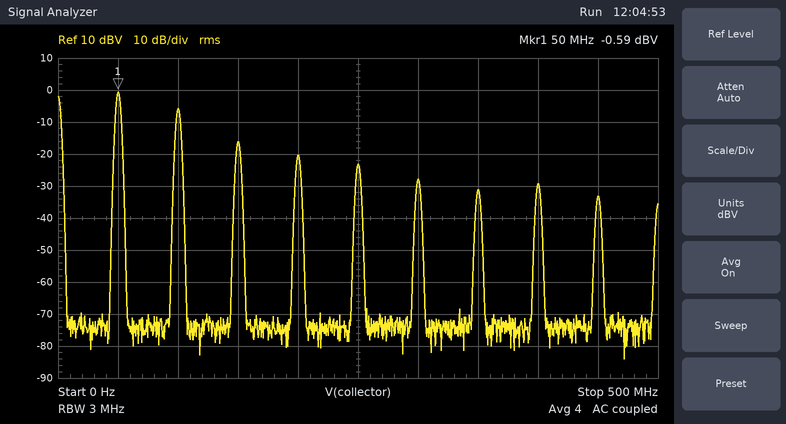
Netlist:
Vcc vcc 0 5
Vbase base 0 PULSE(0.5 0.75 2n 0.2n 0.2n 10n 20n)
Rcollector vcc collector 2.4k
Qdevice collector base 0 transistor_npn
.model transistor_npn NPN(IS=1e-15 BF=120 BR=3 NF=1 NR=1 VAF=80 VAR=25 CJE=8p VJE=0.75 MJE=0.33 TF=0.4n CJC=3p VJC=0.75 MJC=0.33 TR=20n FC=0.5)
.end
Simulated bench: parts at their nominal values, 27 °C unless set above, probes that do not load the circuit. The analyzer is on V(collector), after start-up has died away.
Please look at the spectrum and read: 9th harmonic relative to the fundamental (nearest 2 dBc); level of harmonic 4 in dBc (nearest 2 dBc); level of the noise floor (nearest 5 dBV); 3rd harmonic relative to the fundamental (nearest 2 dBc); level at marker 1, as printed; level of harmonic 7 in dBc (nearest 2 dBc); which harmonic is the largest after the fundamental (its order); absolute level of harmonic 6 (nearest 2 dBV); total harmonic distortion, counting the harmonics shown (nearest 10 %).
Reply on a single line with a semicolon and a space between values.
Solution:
-32 dBc; -20 dBc; -75 dBV; -16 dBc; -0.59 dBV; -30 dBc; 2; -28 dBV; 60 %
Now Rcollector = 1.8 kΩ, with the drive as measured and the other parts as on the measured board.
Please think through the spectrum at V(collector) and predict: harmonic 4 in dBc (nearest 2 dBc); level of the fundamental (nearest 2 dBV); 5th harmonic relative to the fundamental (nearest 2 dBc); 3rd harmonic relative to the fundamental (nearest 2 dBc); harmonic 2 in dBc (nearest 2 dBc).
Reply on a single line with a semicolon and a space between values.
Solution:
-22 dBc; 4 dBV; -30 dBc; -20 dBc; -12 dBc
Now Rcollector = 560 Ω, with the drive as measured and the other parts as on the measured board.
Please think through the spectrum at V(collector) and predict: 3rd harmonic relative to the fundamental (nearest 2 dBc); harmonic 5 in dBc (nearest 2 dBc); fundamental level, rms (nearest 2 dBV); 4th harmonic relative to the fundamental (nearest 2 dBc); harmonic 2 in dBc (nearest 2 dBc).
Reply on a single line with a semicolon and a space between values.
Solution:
-12 dBc; -18 dBc; 0 dBV; -38 dBc; -36 dBc
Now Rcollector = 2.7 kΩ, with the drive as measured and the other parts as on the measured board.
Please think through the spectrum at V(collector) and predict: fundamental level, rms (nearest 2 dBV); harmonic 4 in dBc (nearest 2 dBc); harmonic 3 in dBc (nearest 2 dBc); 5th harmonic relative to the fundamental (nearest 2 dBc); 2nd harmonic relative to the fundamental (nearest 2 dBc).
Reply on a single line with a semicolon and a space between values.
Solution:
-4 dBV; -16 dBc; -10 dBc; -20 dBc; -4 dBc
